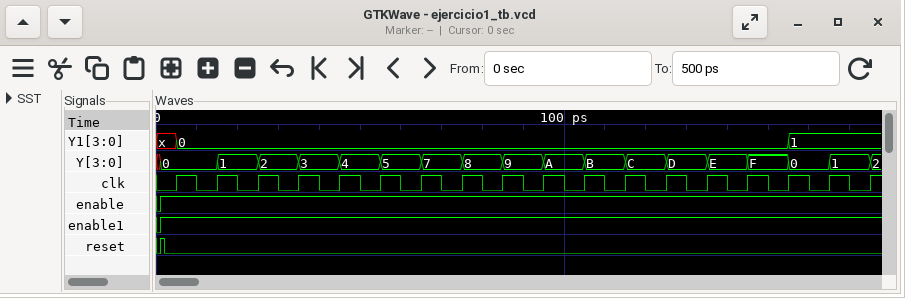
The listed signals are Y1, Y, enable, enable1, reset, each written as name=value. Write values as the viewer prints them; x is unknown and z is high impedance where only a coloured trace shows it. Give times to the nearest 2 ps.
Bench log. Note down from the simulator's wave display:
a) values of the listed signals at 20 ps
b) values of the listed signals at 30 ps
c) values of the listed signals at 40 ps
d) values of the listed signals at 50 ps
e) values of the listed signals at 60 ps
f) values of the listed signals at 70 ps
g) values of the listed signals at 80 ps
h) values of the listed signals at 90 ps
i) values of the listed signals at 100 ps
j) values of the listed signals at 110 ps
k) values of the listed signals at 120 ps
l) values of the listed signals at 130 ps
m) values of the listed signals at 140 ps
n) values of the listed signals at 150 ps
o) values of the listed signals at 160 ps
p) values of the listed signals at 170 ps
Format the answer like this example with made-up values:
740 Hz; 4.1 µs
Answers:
Y1=0, Y=1, enable=1, enable1=1, reset=0; Y1=0, Y=2, enable=1, enable1=1, reset=0; Y1=0, Y=3, enable=1, enable1=1, reset=0; Y1=0, Y=4, enable=1, enable1=1, reset=0; Y1=0, Y=5, enable=1, enable1=1, reset=0; Y1=0, Y=7, enable=1, enable1=1, reset=0; Y1=0, Y=8, enable=1, enable1=1, reset=0; Y1=0, Y=9, enable=1, enable1=1, reset=0; Y1=0, Y=A, enable=1, enable1=1, reset=0; Y1=0, Y=B, enable=1, enable1=1, reset=0; Y1=0, Y=C, enable=1, enable1=1, reset=0; Y1=0, Y=D, enable=1, enable1=1, reset=0; Y1=0, Y=E, enable=1, enable1=1, reset=0; Y1=0, Y=F, enable=1, enable1=1, reset=0; Y1=1, Y=0, enable=1, enable1=1, reset=0; Y1=1, Y=1, enable=1, enable1=1, reset=0
